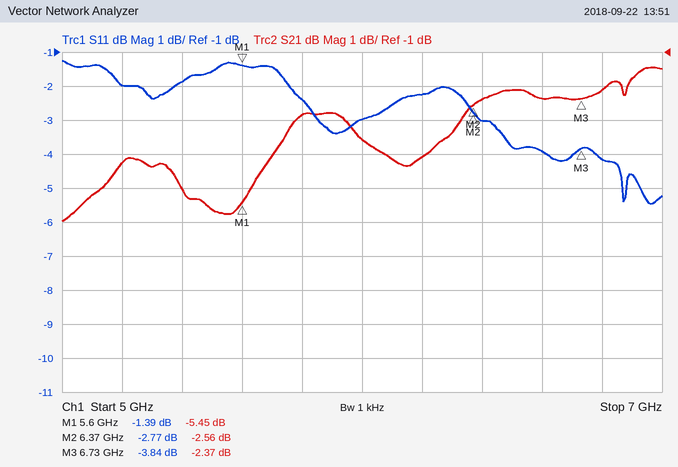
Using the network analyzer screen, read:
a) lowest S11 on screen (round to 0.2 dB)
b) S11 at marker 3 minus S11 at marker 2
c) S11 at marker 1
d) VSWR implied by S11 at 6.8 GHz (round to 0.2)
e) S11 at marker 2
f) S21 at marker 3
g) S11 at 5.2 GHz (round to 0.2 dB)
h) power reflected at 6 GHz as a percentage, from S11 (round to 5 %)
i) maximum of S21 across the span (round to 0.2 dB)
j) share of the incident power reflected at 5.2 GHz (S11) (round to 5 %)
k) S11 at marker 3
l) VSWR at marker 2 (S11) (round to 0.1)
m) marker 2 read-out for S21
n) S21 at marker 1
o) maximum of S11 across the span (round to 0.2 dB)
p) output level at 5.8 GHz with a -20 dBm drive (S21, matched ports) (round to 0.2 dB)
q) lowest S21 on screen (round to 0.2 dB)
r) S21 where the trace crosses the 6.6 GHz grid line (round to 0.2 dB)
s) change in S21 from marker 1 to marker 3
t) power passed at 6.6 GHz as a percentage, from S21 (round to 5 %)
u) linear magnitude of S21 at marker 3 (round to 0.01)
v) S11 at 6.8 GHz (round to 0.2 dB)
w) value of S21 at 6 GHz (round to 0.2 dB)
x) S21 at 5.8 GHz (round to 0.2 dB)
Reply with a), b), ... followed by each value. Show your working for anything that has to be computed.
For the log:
a) -5.4 dB
b) -3.84 − (-2.77) = -1.07 dB
c) -1.39 dB
d) |Γ| = 10^(-4.2/20) = 0.6166; VSWR = (1 + 0.6166)/(1 − 0.6166) ≈ 4.2
e) -2.77 dB
f) -2.37 dB
g) -2.0 dB
h) 10^(-3/10) ≈ 50 %
i) -1.4 dB
j) 10^(-2/10) ≈ 63.1 %, so 65 % to the nearest 5 %
k) -3.84 dB
l) (1 + 0.7269)/(1 − 0.7269) ≈ 6.3
m) -2.56 dB
n) -5.45 dB
o) -1.2 dB
p) -20 dBm + (-2.8 dB) = -22.8 dBm
q) -6.0 dB
r) -2.4 dB
s) -2.37 − (-5.45) = 3.08 dB
t) 10^(-2.4/10) ≈ 57.5 %, so 60 % to the nearest 5 %
u) 10^(-2.37/20) ≈ 0.76
v) -4.2 dB
w) -3.6 dB
x) -2.8 dB
